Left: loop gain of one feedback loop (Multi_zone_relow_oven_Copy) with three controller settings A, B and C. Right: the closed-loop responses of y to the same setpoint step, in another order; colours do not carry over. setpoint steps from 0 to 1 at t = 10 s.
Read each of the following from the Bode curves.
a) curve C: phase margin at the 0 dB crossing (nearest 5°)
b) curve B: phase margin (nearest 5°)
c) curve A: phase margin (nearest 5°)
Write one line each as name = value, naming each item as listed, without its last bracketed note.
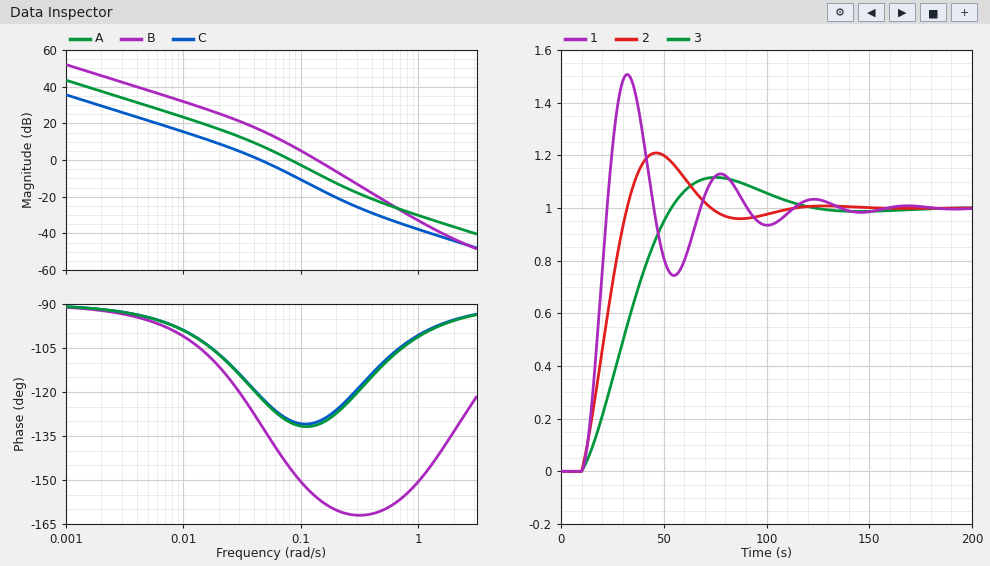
curve C: phase margin at the 0 dB crossing = 60°
curve B: phase margin = 25°
curve A: phase margin = 50°
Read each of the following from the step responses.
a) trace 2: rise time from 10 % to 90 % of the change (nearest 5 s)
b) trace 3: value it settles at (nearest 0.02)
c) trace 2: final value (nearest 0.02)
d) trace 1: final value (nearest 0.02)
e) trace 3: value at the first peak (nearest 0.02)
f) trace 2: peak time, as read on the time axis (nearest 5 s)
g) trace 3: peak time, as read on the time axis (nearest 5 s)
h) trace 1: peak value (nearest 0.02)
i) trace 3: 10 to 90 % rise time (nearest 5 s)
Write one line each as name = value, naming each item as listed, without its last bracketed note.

trace 2: rise time from 10 % to 90 % of the change = 15 s
trace 3: value it settles at = 1.00
trace 2: final value = 1.00
trace 1: final value = 1.00
trace 3: value at the first peak = 1.12
trace 2: peak time, as read on the time axis = 45 s
trace 3: peak time, as read on the time axis = 75 s
trace 1: peak value = 1.50
trace 3: 10 to 90 % rise time = 30 s
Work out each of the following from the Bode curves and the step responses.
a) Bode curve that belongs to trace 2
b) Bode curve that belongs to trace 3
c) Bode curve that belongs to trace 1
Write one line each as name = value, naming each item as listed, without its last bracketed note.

Bode curve that belongs to trace 2 = A
Bode curve that belongs to trace 3 = C
Bode curve that belongs to trace 1 = B
